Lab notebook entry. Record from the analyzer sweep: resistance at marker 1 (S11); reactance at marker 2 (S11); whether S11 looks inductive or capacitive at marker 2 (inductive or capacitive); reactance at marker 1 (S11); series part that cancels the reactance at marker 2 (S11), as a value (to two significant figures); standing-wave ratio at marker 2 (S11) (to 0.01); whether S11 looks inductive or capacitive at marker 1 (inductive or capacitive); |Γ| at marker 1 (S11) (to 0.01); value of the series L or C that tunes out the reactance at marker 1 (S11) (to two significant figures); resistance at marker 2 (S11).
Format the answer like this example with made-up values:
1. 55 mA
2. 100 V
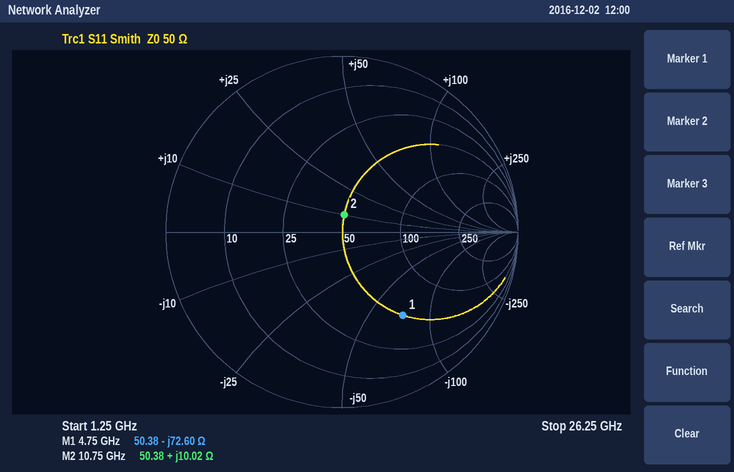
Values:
1. 50.38 Ω
2. +10.02 Ω
3. inductive
4. -72.60 Ω
5. 1.5 pF
6. 1.22
7. capacitive
8. 0.59
9. 2.4 nH
10. 50.38 Ω
